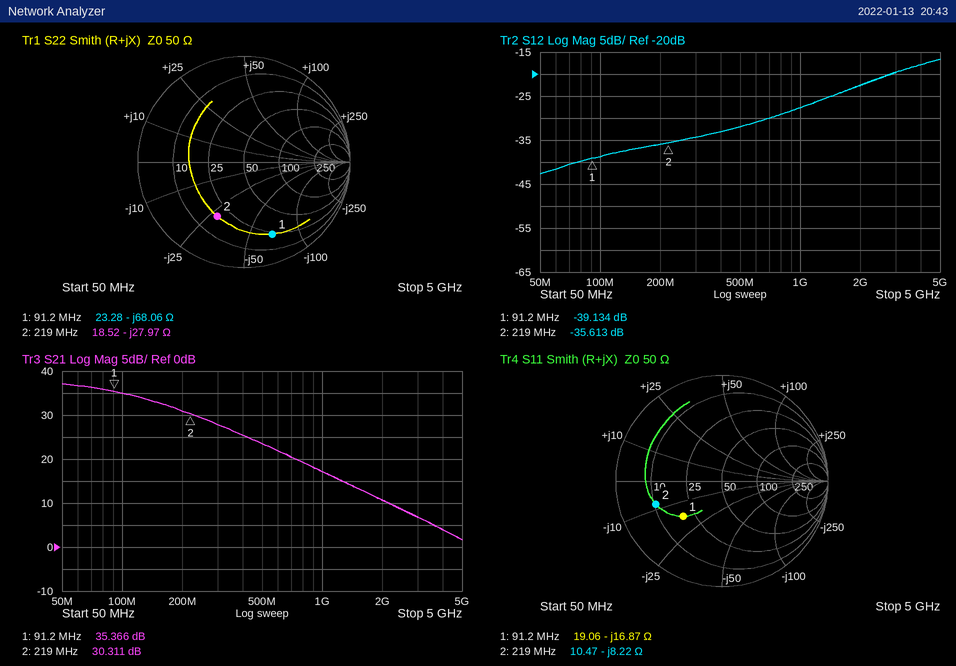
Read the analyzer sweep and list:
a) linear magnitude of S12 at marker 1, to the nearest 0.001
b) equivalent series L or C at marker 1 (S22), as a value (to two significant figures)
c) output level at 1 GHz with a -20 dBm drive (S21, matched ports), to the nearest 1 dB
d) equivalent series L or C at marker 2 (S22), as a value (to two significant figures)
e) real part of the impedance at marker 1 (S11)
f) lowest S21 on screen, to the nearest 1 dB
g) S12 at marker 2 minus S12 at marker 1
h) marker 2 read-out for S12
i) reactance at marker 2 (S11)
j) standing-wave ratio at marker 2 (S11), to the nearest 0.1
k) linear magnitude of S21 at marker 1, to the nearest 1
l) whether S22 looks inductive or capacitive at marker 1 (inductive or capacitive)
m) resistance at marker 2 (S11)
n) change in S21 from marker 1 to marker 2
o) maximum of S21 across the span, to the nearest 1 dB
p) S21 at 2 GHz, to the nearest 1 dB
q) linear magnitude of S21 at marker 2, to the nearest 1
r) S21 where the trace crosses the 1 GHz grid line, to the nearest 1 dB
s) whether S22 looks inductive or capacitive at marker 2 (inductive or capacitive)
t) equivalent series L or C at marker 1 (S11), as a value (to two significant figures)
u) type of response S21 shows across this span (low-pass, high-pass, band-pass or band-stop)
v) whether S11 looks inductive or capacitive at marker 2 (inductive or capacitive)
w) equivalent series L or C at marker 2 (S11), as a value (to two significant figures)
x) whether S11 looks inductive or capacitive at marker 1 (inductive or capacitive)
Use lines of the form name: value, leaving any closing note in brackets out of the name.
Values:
linear magnitude of S12 at marker 1, to the nearest 0.001: 0.011
equivalent series L or C at marker 1 (S22), as a value: 26 pF
output level at 1 GHz with a -20 dBm drive (S21, matched ports), to the nearest 1 dB: -3 dBm
equivalent series L or C at marker 2 (S22), as a value: 26 pF
real part of the impedance at marker 1: 19.06 Ω
lowest S21 on screen, to the nearest 1 dB: 2 dB
S12 at marker 2 minus S12 at marker 1: 3.521 dB
marker 2 read-out for S12: -35.613 dB
reactance at marker 2: -8.22 Ω
standing-wave ratio at marker 2 (S11), to the nearest 0.1: 4.9
linear magnitude of S21 at marker 1, to the nearest 1: 59
whether S22 looks inductive or capacitive at marker 1: capacitive
resistance at marker 2: 10.47 Ω
change in S21 from marker 1 to marker 2: -5.055 dB
maximum of S21 across the span, to the nearest 1 dB: 37 dB
S21 at 2 GHz, to the nearest 1 dB: 11 dB
linear magnitude of S21 at marker 2, to the nearest 1: 33
S21 where the trace crosses the 1 GHz grid line, to the nearest 1 dB: 17 dB
whether S22 looks inductive or capacitive at marker 2: capacitive
equivalent series L or C at marker 1 (S11), as a value: 100 pF
type of response S21 shows across this span: low-pass
whether S11 looks inductive or capacitive at marker 2: capacitive
equivalent series L or C at marker 2 (S11), as a value: 88 pF
whether S11 looks inductive or capacitive at marker 1: capacitive
